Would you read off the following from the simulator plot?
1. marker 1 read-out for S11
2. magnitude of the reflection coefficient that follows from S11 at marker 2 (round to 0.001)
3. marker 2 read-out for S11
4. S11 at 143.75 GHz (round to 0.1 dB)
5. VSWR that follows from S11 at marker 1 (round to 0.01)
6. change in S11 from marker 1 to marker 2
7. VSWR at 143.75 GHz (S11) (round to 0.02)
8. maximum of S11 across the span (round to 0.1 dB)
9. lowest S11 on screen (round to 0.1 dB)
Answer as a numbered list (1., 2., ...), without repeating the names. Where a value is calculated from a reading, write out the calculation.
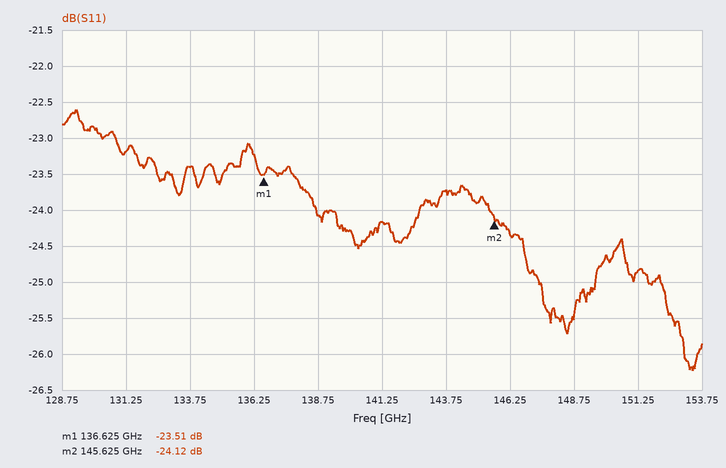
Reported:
1. -23.51 dB
2. 10^(-24.12/20) ≈ 0.062
3. -24.12 dB
4. -23.7 dB
5. (1 + 0.0668)/(1 − 0.0668) ≈ 1.14
6. -24.12 − (-23.51) = -0.61 dB
7. |Γ| = 10^(-23.7/20) = 0.0653; VSWR = (1 + 0.0653)/(1 − 0.0653) ≈ 1.14
8. -22.6 dB
9. -26.2 dB
